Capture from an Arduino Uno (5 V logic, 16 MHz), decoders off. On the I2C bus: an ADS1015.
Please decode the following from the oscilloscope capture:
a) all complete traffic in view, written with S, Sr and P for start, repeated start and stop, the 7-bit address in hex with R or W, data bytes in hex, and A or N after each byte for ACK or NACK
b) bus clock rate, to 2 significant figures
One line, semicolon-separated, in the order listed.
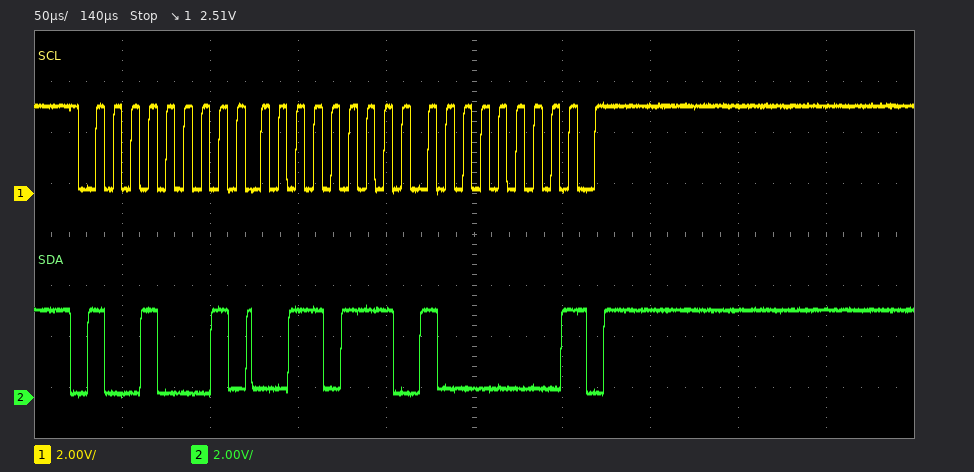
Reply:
S 48R A 37 A 80 N P; 100 kHz
